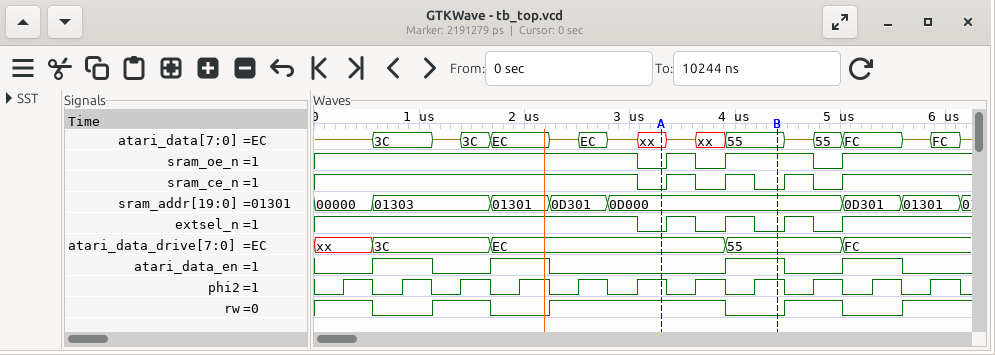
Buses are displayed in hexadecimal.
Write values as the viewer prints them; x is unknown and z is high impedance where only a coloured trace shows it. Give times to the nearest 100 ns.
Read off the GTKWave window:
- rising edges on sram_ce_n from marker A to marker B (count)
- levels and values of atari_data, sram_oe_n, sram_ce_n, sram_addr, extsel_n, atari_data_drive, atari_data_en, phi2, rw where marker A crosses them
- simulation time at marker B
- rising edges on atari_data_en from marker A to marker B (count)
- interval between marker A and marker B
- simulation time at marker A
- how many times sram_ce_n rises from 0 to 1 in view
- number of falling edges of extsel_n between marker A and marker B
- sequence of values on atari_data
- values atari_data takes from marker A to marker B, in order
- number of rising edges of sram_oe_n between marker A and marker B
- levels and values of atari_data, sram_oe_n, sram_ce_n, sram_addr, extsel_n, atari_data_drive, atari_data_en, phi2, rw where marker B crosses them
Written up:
2
atari_data=xx, sram_oe_n=0, sram_ce_n=0, sram_addr=0D000, extsel_n=0, atari_data_drive=EC, atari_data_en=0, phi2=1, rw=1
4400 ns
1
1100 ns
3300 ns
4
2
z, 3C, z, 3C, EC, z, EC, z, xx, z, xx, 55, z, 55, FC, z, FC, z
xx, z, xx, 55
2
atari_data=55, sram_oe_n=1, sram_ce_n=0, sram_addr=0D000, extsel_n=0, atari_data_drive=55, atari_data_en=1, phi2=1, rw=0
